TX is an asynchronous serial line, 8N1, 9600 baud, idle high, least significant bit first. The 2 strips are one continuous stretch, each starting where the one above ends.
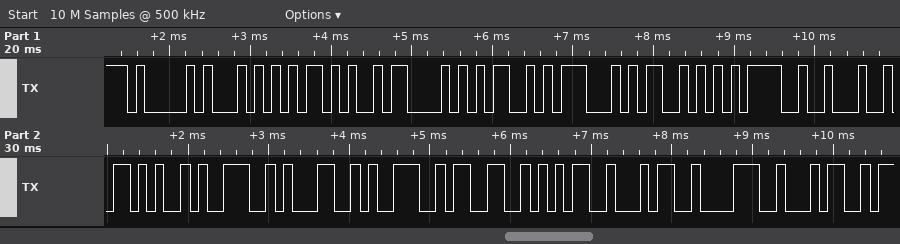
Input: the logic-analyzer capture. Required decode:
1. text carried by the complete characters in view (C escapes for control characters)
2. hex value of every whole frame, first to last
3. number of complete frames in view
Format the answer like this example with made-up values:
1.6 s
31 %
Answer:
"AT+CMGS=\"+91935484"
41 54 2B 43 4D 47 53 3D 22 2B 39 31 39 33 35 34 38 34
18
